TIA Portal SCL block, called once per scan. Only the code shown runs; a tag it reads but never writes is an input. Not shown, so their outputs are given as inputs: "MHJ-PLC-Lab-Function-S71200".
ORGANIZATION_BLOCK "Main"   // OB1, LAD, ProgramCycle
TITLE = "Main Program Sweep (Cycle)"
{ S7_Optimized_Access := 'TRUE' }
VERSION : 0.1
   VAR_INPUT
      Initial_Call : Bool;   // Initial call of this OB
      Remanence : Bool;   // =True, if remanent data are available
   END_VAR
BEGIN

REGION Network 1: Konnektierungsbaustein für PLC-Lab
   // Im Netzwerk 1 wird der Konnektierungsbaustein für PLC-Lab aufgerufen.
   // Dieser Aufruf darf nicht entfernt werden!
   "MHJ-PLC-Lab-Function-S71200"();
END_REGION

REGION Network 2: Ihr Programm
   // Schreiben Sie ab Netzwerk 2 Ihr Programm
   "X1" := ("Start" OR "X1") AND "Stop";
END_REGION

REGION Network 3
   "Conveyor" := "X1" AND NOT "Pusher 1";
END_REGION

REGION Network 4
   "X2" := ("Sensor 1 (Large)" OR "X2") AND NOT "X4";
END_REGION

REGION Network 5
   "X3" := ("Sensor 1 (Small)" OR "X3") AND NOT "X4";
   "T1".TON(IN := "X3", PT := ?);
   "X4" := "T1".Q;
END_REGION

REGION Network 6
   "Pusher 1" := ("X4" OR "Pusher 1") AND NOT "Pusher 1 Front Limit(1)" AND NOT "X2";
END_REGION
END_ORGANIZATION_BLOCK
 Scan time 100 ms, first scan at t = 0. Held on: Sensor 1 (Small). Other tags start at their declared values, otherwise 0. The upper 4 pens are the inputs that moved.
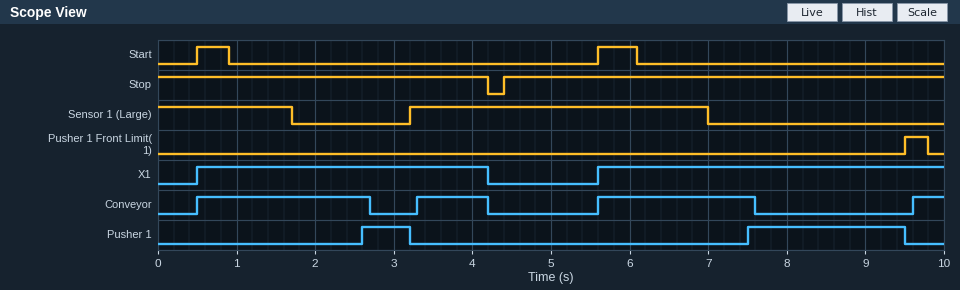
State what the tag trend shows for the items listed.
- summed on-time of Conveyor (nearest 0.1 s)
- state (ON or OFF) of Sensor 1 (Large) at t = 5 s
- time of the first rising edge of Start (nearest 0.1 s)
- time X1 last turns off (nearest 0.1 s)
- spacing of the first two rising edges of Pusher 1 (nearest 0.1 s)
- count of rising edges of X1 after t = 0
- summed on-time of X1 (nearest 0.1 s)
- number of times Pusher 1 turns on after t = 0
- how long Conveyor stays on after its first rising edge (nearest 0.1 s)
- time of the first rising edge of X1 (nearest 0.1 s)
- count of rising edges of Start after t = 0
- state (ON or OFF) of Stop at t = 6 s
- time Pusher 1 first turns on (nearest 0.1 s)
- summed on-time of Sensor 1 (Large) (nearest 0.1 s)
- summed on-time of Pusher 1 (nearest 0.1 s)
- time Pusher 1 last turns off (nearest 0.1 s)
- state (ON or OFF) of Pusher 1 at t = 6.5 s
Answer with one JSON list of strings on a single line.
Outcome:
["5.5 s", "ON", "0.5 s", "4.2 s", "4.9 s", "2", "8.1 s", "2", "2.2 s", "0.5 s", "2", "ON", "2.6 s", "5.5 s", "2.6 s", "9.5 s", "OFF"]
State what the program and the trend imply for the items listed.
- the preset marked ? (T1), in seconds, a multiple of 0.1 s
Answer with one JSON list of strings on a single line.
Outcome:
["0.5 s"]
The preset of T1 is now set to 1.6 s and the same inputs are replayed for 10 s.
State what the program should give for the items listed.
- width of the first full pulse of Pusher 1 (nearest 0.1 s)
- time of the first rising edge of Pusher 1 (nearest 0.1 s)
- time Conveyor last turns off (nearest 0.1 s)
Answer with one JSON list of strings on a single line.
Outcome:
["0.7 s", "8.8 s", "8.9 s"]
